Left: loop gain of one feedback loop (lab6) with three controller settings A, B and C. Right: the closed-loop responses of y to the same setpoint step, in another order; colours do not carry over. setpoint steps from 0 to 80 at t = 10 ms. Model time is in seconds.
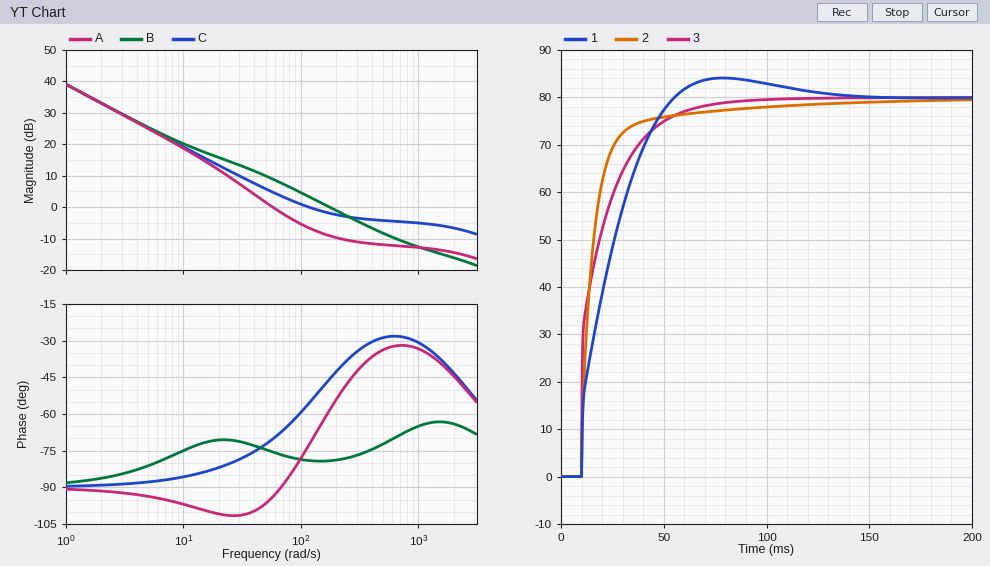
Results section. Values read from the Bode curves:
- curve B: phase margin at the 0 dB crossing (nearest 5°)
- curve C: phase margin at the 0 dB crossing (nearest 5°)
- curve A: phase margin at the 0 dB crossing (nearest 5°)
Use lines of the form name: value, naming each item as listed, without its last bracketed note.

curve B: phase margin at the 0 dB crossing: 100°
curve C: phase margin at the 0 dB crossing: 125°
curve A: phase margin at the 0 dB crossing: 85°
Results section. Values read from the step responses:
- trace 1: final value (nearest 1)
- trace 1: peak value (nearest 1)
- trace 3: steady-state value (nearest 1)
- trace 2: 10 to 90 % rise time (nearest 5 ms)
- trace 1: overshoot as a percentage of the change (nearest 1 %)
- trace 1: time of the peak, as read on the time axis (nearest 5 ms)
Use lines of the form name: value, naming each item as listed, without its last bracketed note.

trace 1: final value: 80
trace 1: peak value: 84
trace 3: steady-state value: 80
trace 2: 10 to 90 % rise time: 20 ms
trace 1: overshoot as a percentage of the change: 5 %
trace 1: time of the peak, as read on the time axis: 80 ms
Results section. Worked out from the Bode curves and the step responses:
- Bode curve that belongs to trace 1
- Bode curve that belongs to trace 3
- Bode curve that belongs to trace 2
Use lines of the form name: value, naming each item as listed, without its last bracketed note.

Bode curve that belongs to trace 1: A
Bode curve that belongs to trace 3: C
Bode curve that belongs to trace 2: B
